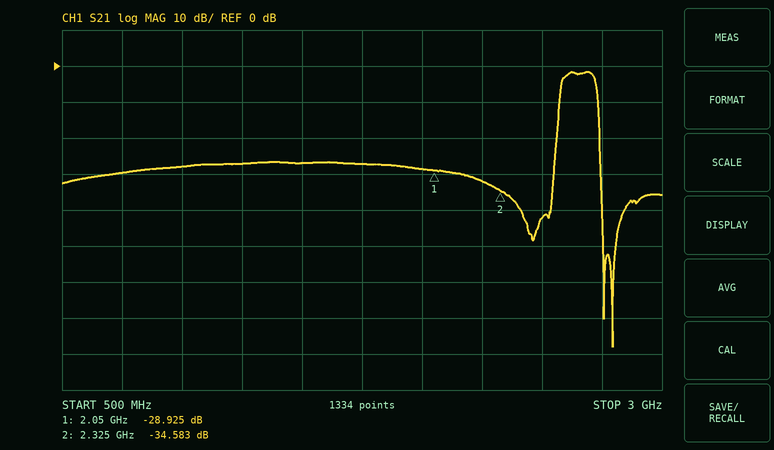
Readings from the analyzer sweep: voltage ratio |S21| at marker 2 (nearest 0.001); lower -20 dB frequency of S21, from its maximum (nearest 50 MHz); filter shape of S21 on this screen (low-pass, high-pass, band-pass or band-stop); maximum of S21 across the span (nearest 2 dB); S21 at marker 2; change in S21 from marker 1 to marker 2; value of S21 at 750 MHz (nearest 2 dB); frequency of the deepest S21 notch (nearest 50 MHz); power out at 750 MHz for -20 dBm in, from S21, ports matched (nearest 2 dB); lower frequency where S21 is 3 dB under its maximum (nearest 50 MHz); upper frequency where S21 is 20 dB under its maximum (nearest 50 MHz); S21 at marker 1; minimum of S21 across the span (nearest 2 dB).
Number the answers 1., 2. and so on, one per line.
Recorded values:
1. 0.019
2. 2.55 GHz
3. band-pass
4. -2 dB
5. -34.583 dB
6. -5.658 dB
7. -30 dB
8. 2.80 GHz
9. -50 dBm
10. 2.60 GHz
11. 2.75 GHz
12. -28.925 dB
13. -78 dB
